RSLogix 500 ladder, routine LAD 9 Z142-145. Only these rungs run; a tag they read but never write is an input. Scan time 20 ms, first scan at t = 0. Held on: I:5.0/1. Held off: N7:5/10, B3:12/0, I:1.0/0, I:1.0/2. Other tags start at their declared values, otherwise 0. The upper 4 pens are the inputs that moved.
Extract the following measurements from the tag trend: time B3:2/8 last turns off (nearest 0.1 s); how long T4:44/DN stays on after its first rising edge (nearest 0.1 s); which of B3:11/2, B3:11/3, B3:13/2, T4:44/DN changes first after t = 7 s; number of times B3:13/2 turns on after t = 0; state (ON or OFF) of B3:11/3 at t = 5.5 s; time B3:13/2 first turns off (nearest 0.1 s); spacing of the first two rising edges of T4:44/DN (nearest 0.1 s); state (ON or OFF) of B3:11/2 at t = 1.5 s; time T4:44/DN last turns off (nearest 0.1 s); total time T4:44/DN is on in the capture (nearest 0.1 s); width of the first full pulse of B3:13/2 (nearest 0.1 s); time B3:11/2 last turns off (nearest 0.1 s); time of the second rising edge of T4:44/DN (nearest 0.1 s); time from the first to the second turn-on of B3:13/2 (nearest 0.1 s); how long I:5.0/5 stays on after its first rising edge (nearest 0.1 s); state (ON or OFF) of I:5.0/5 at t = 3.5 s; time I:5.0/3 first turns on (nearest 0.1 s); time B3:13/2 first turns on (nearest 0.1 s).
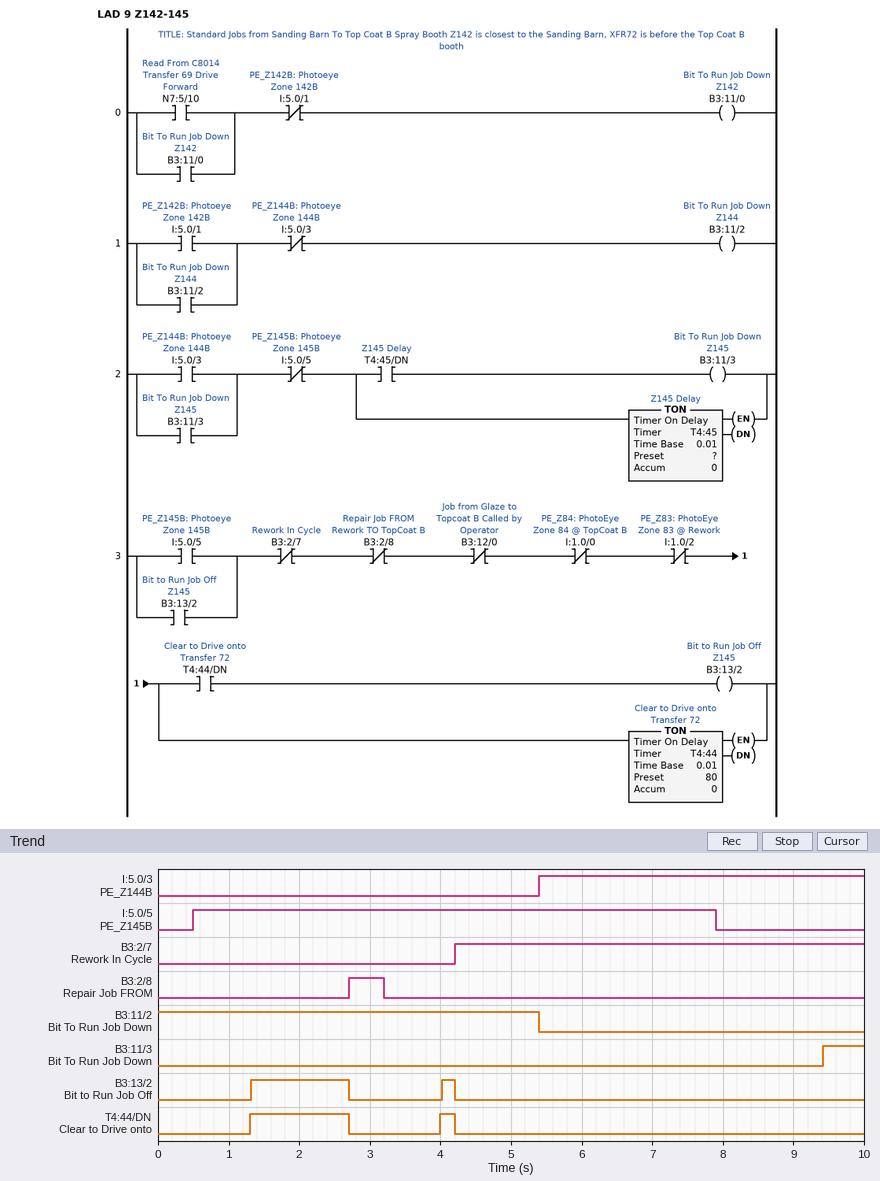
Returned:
3.2 s
1.4 s
B3:11/3
2
OFF
2.7 s
2.7 s
ON
4.2 s
1.6 s
1.4 s
5.4 s
4.0 s
2.7 s
7.4 s
ON
5.4 s
1.3 s
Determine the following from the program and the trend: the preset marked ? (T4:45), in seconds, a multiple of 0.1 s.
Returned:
1.5 s
